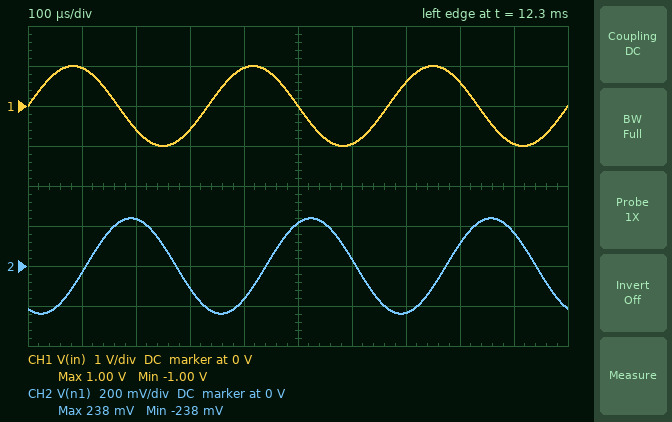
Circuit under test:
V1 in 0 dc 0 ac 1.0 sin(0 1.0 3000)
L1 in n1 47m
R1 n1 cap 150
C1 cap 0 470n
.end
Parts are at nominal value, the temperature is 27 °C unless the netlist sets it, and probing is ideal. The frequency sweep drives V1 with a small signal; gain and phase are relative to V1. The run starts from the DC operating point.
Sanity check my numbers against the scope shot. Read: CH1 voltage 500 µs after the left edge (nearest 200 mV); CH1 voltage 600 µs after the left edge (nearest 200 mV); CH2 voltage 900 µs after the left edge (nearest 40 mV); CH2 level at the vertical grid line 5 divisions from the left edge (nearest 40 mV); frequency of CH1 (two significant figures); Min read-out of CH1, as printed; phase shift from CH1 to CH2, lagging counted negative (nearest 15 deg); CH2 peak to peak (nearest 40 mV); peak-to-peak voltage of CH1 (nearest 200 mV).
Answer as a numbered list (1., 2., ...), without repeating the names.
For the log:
1. 0 V
2. -1.0 V
3. 160 mV
4. 200 mV
5. 3.0 kHz
6. -1.00 V
7. -120 deg
8. 480 mV
9. 2.0 V
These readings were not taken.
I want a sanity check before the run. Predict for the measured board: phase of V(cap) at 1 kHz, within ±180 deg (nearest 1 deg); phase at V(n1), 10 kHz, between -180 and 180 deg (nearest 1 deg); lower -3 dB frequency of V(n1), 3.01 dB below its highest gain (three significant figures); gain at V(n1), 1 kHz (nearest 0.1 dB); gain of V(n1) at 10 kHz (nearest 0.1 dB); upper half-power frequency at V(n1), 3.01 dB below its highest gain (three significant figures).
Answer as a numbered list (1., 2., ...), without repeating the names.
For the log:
1. -74 deg
2. -100 deg
3. 731 Hz
4. 7.5 dB
5. -25.6 dB
6. 1.26 kHz
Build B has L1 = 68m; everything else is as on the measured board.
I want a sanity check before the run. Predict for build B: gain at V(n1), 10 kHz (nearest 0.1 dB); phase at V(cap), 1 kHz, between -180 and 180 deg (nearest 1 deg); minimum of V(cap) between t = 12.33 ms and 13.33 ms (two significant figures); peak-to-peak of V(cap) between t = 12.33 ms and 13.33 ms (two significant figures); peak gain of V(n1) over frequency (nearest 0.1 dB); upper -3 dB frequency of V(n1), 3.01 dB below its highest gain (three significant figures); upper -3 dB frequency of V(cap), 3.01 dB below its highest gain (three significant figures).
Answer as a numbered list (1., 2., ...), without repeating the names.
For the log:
1. -28.8 dB
2. -121 deg
3. -96 mV
4. 190 mV
5. 8.8 dB
6. 1.03 kHz
7. 1.02 kHz
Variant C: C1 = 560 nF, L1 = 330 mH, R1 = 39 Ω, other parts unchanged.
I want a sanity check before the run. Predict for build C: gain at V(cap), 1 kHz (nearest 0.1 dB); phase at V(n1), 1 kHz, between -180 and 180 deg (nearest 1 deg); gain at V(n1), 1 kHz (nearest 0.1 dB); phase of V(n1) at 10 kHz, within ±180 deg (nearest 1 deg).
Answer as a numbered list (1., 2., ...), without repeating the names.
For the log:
1. -16.0 dB
2. -171 deg
3. -15.9 dB
4. -126 deg
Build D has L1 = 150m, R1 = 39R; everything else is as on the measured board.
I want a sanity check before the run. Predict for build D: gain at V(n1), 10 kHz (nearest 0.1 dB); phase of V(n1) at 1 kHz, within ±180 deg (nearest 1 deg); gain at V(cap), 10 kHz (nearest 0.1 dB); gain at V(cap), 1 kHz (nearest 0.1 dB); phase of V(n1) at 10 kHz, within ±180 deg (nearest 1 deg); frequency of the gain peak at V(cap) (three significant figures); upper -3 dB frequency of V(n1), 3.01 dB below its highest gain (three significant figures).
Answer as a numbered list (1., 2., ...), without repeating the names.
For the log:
1. -45.2 dB
2. -170 deg
3. -48.9 dB
4. -5.0 dB
5. -131 deg
6. 599 Hz
7. 619 Hz
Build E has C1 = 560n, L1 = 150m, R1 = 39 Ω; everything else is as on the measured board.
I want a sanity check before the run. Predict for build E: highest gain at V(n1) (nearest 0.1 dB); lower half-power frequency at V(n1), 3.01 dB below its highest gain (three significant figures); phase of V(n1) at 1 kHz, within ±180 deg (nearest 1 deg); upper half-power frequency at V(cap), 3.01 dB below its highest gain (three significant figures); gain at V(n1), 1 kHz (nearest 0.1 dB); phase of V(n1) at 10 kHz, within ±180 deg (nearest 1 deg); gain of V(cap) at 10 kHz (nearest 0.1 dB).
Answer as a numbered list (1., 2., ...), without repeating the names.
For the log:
1. 22.5 dB
2. 527 Hz
3. -169 deg
4. 569 Hz
5. -7.2 dB
6. -126 deg
7. -50.4 dB
